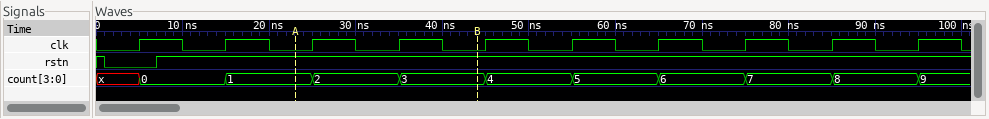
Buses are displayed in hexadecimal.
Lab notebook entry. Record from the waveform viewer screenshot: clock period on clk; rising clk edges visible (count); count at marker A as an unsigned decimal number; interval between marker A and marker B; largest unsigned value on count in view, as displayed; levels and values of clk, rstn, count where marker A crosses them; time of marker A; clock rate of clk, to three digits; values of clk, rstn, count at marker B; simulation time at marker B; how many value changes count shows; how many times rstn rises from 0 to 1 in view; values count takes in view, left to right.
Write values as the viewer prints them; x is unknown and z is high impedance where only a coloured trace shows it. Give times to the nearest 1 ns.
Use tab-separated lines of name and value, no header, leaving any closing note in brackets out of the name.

clock period on clk	10 ns
rising clk edges visible	10
count at marker A as an unsigned decimal number	1
interval between marker A and marker B	21 ns
largest unsigned value on count in view, as displayed	9
levels and values of clk, rstn, count where marker A crosses them	clk=0, rstn=1, count=1
time of marker A	23 ns
clock rate of clk, to three digits	100 MHz
values of clk, rstn, count at marker B	clk=0, rstn=1, count=3
simulation time at marker B	44 ns
how many value changes count shows	10
how many times rstn rises from 0 to 1 in view	1
values count takes in view, left to right	x, 0, 1, 2, 3, 4, 5, 6, 7, 8, 9
